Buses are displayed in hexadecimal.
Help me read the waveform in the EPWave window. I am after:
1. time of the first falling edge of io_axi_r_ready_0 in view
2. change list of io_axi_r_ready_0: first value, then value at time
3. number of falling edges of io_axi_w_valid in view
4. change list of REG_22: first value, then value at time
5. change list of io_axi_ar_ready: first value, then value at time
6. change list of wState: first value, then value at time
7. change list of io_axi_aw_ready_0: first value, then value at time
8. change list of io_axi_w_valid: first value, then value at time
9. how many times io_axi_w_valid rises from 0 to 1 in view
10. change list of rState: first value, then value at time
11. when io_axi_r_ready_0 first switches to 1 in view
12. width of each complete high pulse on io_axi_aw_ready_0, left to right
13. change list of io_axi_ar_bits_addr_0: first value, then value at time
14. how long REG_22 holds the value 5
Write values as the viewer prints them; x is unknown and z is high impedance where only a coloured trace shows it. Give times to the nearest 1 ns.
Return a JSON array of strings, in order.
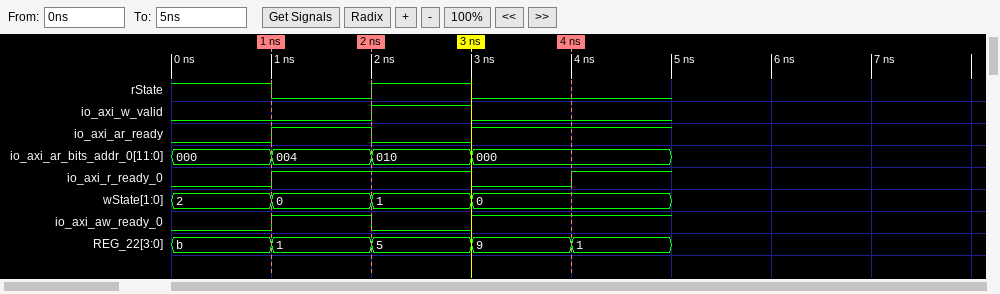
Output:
["3 ns", "0, 1 at 1 ns, 0 at 3 ns, 1 at 4 ns", "1", "b, 1 at 1 ns, 5 at 2 ns, 9 at 3 ns, 1 at 4 ns", "0, 1 at 1 ns, 0 at 2 ns, 1 at 3 ns", "2, 0 at 1 ns, 1 at 2 ns, 0 at 3 ns", "0, 1 at 1 ns, 0 at 2 ns, 1 at 3 ns", "0, 1 at 2 ns, 0 at 3 ns", "1", "1, 0 at 1 ns, 1 at 2 ns, 0 at 3 ns", "1 ns", "1 ns", "000, 004 at 1 ns, 010 at 2 ns, 000 at 3 ns", "1 ns"]
